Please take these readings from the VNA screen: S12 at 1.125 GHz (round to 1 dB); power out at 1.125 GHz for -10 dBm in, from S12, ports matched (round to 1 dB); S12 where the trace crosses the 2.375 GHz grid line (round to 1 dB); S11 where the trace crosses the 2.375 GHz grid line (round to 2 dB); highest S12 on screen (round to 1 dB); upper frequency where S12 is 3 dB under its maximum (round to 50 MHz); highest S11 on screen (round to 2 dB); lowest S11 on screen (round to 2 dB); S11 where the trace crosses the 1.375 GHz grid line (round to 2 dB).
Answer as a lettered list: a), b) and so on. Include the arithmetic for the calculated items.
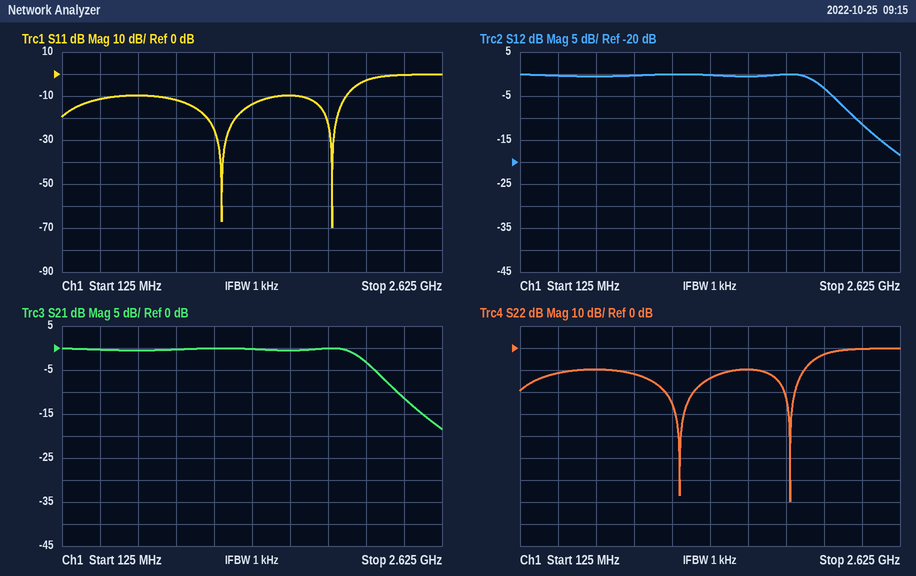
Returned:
a) 0 dB
b) -10 dBm + (0 dB) = -10 dBm
c) -11 dB
d) 0 dB
e) 0 dB
f) 2.10 GHz
g) 0 dB
h) -70 dB
i) -14 dB
